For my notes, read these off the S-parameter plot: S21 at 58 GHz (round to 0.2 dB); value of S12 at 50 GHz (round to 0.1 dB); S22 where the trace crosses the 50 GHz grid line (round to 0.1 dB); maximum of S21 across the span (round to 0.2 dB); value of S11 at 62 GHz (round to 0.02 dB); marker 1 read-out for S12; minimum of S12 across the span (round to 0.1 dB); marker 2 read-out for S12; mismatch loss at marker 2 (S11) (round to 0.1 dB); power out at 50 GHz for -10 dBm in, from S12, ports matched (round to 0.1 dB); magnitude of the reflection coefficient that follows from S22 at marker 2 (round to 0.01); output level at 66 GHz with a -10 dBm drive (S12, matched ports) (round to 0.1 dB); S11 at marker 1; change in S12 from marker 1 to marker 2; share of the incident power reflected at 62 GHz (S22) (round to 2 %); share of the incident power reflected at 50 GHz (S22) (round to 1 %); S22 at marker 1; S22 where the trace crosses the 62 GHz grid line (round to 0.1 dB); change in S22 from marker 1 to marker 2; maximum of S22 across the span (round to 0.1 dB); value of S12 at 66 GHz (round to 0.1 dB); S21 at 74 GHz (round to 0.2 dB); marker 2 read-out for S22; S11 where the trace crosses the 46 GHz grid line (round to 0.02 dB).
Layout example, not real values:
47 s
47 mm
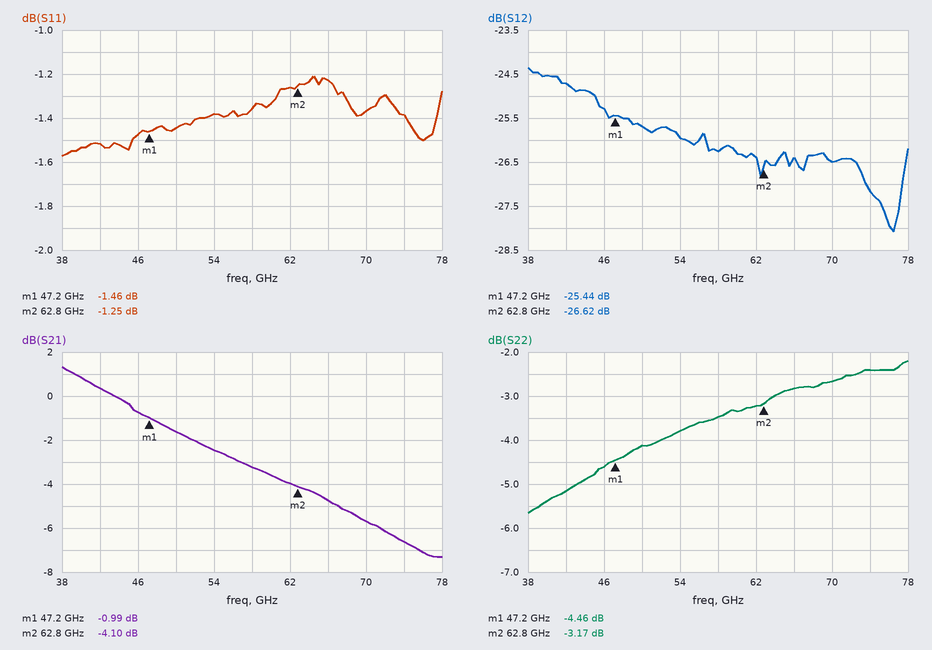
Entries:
-3.2 dB
-25.7 dB
-4.1 dB
1.4 dB
-1.26 dB
-25.44 dB
-28.1 dB
-26.62 dB
6.0 dB
-35.7 dBm
0.69
-36.4 dBm
-1.46 dB
-1.18 dB
48 %
39 %
-4.46 dB
-3.2 dB
1.29 dB
-2.2 dB
-26.4 dB
-6.6 dB
-3.17 dB
-1.48 dB
